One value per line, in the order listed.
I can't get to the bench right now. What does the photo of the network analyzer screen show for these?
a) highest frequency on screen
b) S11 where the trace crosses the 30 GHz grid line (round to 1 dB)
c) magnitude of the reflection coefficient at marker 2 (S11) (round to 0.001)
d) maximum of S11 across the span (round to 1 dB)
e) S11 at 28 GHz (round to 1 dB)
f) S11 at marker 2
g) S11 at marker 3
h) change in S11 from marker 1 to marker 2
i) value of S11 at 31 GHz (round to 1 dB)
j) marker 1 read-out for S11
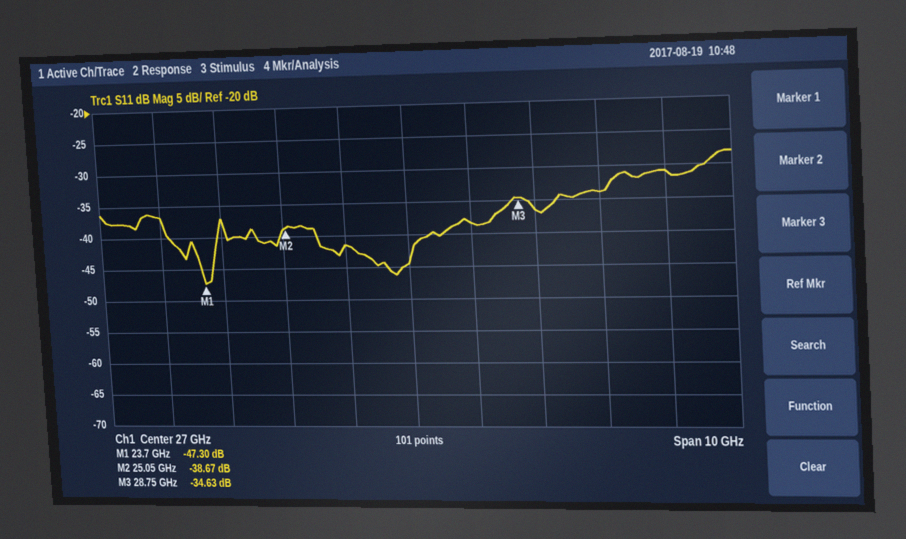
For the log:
32 GHz
-34 dB
0.012
-28 dB
-38 dB
-38.67 dB
-34.63 dB
8.63 dB
-31 dB
-47.30 dB
